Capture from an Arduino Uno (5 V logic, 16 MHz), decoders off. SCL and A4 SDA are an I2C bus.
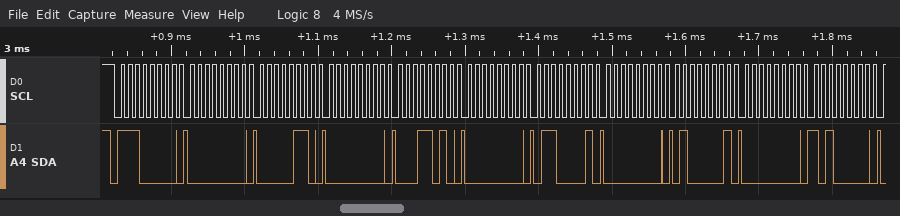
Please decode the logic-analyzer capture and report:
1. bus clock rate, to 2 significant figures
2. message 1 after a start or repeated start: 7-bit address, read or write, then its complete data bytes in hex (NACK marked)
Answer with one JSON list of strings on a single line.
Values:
["100 kHz", "0x70 write: 00 06 00 1A 00 61 00 41 00 A0"]
